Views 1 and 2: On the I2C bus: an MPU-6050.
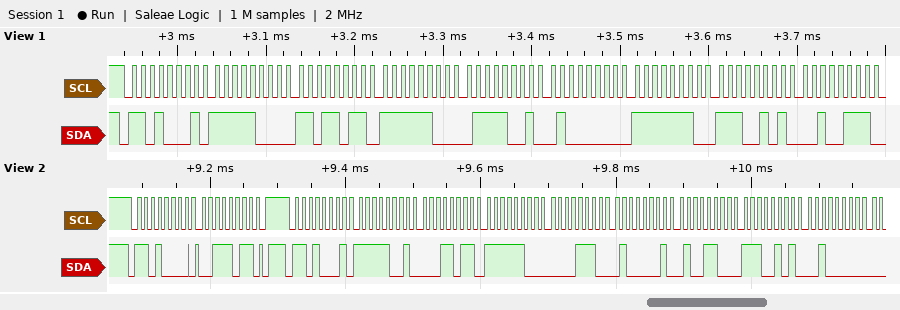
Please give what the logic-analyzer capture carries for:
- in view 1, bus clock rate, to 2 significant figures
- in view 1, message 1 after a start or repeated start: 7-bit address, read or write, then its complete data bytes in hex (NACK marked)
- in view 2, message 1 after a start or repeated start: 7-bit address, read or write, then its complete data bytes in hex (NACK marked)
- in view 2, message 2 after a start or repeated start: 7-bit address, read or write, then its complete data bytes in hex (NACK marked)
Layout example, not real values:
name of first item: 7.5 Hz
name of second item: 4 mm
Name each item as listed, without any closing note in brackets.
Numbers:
in view 1, bus clock rate, to 2 significant figures: 100 kHz
in view 1, message 1 after a start or repeated start: 7-bit address, read or write, then its complete data bytes in hex: 0x68 read: F8 DB FC 79 40 FE E5 27
in view 2, message 1 after a start or repeated start: 7-bit address, read or write, then its complete data bytes in hex: 0x68 write: 3B
in view 2, message 2 after a start or repeated start: 7-bit address, read or write, then its complete data bytes in hex: 0x68 read: F9 1B FC 0E 41 4C E5 20
